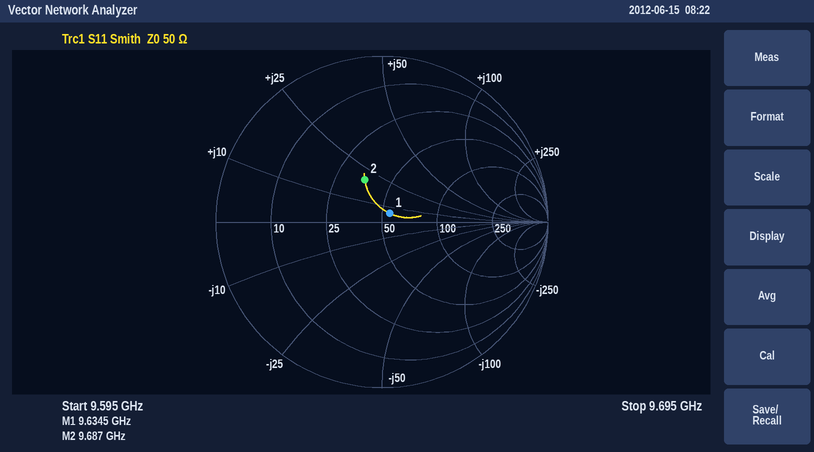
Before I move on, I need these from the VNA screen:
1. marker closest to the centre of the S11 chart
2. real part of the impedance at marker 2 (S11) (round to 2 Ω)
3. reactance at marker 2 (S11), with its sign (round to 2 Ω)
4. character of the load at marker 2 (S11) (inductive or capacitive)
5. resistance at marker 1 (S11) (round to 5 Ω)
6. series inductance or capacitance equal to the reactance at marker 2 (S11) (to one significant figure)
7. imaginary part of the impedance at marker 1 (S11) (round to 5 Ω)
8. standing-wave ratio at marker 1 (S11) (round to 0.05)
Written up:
marker 1
36 Ω
+20 Ω
inductive
55 Ω
300 pH
+5 Ω
1.15
